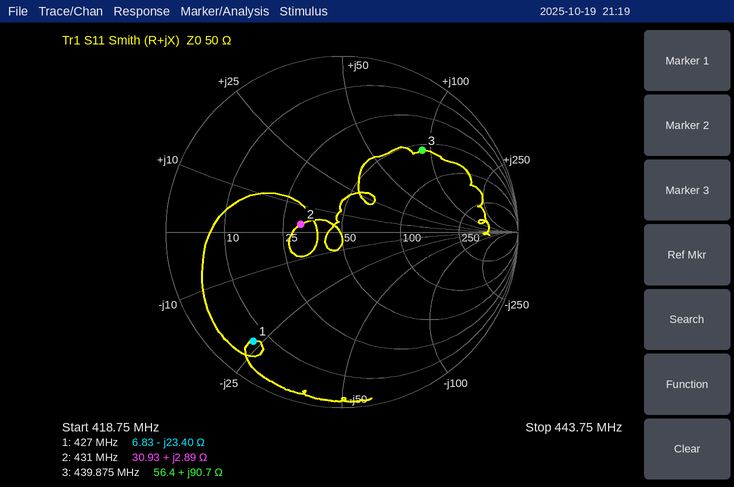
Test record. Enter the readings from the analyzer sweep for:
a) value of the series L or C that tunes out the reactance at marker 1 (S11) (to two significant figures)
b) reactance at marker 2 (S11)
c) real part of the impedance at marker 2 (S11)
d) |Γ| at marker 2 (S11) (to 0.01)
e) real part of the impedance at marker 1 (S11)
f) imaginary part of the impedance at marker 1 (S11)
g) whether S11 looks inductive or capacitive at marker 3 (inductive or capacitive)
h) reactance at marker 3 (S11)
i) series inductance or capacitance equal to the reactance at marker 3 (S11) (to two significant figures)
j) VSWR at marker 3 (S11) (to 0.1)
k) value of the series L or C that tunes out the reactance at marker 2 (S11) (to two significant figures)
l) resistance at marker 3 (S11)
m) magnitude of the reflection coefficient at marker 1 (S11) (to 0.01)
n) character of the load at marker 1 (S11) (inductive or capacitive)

8.7 nH
+2.89 Ω
30.93 Ω
0.24
6.83 Ω
-23.40 Ω
inductive
+90.7 Ω
33 nH
4.7
130 pF
56.4 Ω
0.80
capacitive
